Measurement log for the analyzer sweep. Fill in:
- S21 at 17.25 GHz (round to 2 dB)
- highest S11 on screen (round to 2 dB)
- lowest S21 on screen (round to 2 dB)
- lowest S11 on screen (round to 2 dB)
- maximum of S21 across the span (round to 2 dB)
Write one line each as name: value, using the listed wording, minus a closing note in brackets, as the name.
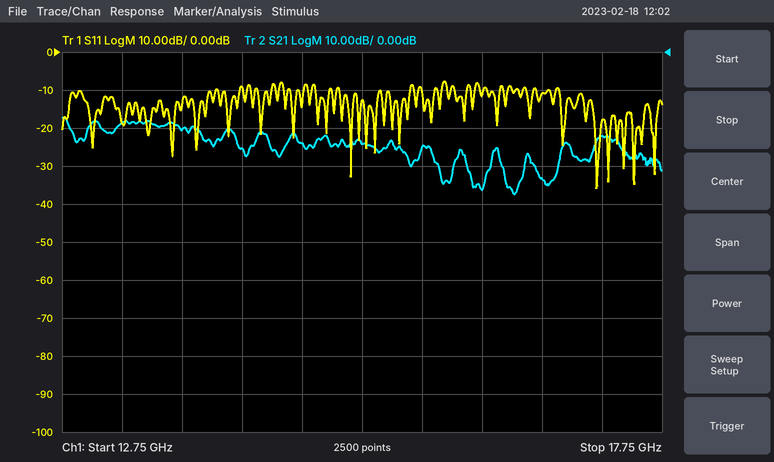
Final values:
S21 at 17.25 GHz: -22 dB
highest S11 on screen: -8 dB
lowest S21 on screen: -38 dB
lowest S11 on screen: -36 dB
maximum of S21 across the span: -18 dB
